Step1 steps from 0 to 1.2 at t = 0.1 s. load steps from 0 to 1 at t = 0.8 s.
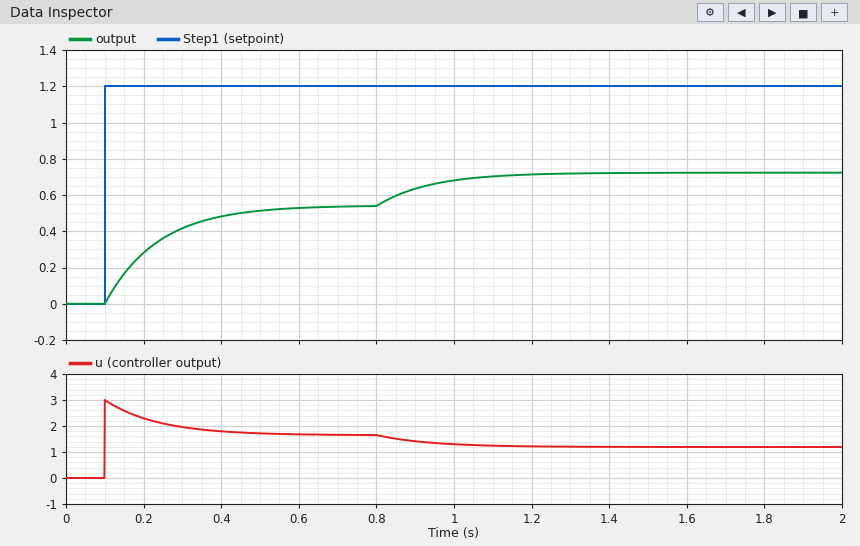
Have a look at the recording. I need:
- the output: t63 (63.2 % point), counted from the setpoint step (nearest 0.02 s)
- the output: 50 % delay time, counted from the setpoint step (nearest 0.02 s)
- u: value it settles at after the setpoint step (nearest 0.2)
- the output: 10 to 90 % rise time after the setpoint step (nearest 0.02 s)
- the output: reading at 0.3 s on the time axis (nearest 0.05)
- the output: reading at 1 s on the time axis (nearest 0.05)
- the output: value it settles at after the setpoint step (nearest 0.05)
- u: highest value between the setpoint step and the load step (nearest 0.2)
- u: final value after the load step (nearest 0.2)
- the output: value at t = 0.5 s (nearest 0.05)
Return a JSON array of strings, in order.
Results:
["0.14 s", "0.10 s", "1.6", "0.30 s", "0.40", "0.70", "0.55", "3.0", "1.2", "0.50"]
